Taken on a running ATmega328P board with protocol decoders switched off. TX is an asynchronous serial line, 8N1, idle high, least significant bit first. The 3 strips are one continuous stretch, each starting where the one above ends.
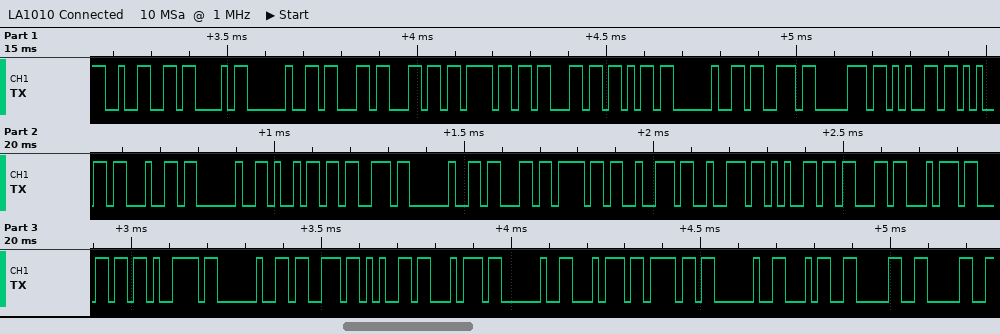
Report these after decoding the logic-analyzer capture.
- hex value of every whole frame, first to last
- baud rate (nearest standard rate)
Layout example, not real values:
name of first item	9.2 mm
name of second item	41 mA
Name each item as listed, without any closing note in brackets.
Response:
hex value of every whole frame, first to last	32 43 20 63 6C 6F 63 6B 20 73 70 65 65 64 20 69 73 20 63 6F 72 72 65 63 74 6C 79 20 73 65 74 20 74 6F 20 34 30 30
baud rate	57600 baud
